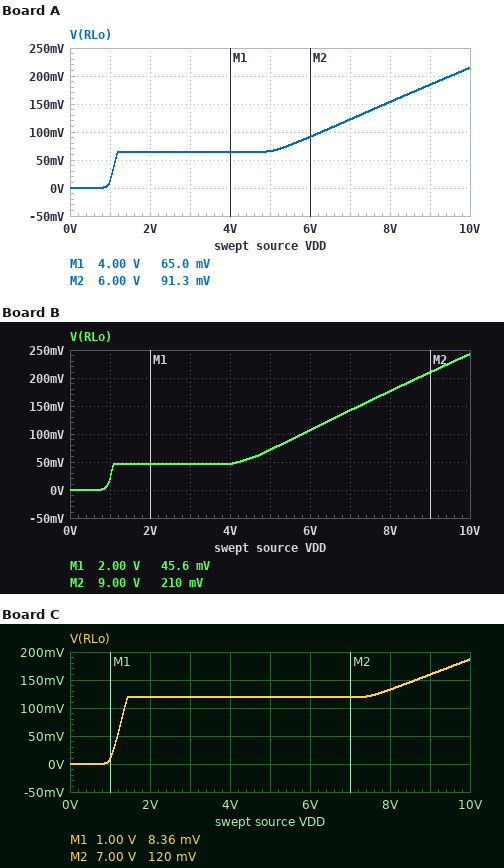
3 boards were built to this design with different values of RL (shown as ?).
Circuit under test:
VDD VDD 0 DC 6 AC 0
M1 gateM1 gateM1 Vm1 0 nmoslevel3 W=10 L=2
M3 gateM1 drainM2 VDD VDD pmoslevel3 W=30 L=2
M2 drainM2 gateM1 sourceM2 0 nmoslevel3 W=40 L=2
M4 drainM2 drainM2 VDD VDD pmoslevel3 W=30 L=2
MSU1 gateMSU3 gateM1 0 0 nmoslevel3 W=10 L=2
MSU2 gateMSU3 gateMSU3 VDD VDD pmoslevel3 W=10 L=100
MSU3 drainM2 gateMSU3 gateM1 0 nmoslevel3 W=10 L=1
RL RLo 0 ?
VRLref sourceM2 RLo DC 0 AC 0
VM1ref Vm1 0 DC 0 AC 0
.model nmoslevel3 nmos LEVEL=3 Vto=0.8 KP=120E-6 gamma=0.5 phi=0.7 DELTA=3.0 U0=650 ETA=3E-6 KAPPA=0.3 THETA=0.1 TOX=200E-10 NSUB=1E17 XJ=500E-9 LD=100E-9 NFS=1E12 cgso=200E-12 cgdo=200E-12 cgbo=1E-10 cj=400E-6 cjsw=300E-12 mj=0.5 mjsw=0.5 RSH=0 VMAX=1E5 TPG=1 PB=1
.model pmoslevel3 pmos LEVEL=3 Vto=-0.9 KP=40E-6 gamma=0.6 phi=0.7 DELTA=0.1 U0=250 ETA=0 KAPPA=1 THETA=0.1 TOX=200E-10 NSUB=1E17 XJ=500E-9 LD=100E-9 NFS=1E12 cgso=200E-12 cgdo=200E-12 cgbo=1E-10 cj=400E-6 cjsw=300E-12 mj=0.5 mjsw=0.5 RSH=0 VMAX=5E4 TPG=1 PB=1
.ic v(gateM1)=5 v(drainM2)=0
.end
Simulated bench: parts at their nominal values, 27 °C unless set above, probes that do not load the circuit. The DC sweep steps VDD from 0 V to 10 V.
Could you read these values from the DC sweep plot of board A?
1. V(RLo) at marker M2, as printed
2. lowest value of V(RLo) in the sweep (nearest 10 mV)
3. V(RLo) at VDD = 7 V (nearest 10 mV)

91.3 mV
0 V
120 mV
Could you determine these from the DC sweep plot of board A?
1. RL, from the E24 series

9.1 kΩ
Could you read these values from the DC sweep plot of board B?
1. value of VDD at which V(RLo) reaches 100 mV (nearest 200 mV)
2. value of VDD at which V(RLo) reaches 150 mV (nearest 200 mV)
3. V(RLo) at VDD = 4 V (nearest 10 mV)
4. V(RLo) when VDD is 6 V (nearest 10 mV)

5.8 V
7.2 V
50 mV
110 mV
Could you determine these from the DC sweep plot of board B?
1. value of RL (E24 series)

18 kΩ
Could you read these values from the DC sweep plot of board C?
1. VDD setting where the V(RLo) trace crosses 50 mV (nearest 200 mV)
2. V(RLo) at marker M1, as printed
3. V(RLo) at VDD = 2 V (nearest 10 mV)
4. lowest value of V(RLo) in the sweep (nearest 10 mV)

1.2 V
8.36 mV
120 mV
0 V
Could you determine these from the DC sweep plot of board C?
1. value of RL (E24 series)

5.1 kΩ
